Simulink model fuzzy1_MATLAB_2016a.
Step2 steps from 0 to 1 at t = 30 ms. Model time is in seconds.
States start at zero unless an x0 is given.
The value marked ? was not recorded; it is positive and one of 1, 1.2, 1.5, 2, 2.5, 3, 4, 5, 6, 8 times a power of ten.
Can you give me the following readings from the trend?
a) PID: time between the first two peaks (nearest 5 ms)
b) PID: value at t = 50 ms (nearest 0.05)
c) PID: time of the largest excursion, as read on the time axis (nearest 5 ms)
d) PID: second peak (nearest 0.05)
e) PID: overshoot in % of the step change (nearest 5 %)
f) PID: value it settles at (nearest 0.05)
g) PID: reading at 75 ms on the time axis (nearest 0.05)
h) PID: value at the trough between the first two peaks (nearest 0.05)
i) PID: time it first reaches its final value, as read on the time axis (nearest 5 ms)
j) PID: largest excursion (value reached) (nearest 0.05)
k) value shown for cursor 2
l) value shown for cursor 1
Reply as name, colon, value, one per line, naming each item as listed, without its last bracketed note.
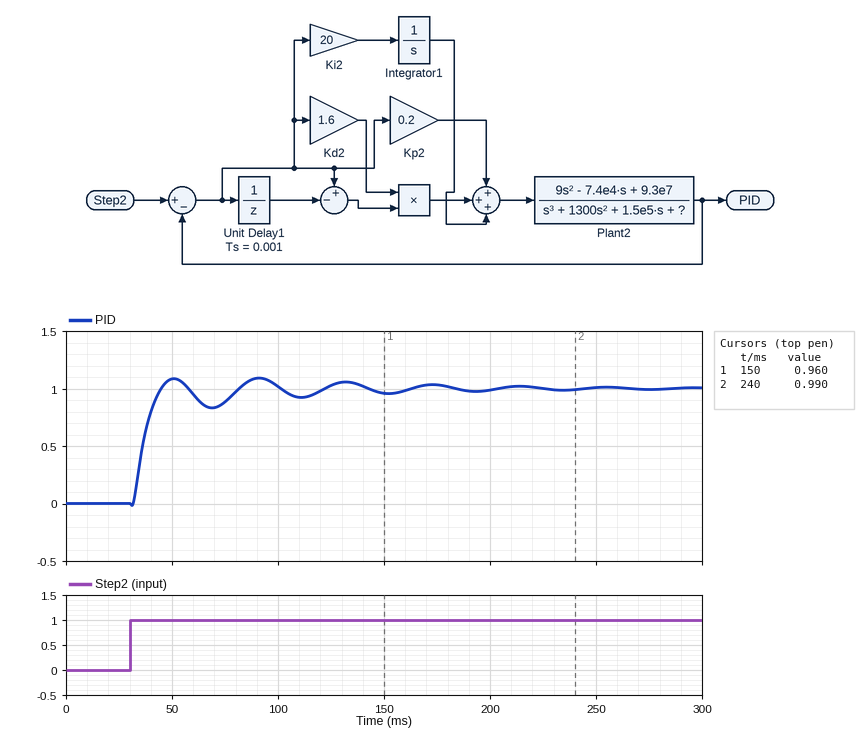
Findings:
PID: time between the first two peaks: 40 ms
PID: value at t = 50 ms: 1.10
PID: time of the largest excursion, as read on the time axis: 90 ms
PID: second peak: 1.10
PID: overshoot in % of the step change: 10 %
PID: value it settles at: 1.00
PID: reading at 75 ms on the time axis: 0.90
PID: value at the trough between the first two peaks: 0.85
PID: time it first reaches its final value, as read on the time axis: 45 ms
PID: largest excursion (value reached): 1.10
value shown for cursor 2: 0.990
value shown for cursor 1: 0.960
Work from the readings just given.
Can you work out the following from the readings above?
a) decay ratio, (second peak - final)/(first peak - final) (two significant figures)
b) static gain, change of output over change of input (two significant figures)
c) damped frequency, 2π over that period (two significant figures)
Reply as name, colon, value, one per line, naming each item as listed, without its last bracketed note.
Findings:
decay ratio, (second peak - final)/(first peak - final): 1.0
static gain, change of output over change of input: 1.0
damped frequency, 2π over that period: 0.16 rad/ms
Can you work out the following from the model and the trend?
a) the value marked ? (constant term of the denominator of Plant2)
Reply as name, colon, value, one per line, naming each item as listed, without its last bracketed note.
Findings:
the value marked ?: 1.5e+07
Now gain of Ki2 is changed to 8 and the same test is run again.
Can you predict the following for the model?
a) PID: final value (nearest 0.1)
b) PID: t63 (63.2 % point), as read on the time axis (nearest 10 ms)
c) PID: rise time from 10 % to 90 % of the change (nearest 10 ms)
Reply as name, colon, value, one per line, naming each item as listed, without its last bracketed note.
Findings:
PID: final value: 1.0
PID: t63 (63.2 % point), as read on the time axis: 40 ms
PID: rise time from 10 % to 90 % of the change: 50 ms
